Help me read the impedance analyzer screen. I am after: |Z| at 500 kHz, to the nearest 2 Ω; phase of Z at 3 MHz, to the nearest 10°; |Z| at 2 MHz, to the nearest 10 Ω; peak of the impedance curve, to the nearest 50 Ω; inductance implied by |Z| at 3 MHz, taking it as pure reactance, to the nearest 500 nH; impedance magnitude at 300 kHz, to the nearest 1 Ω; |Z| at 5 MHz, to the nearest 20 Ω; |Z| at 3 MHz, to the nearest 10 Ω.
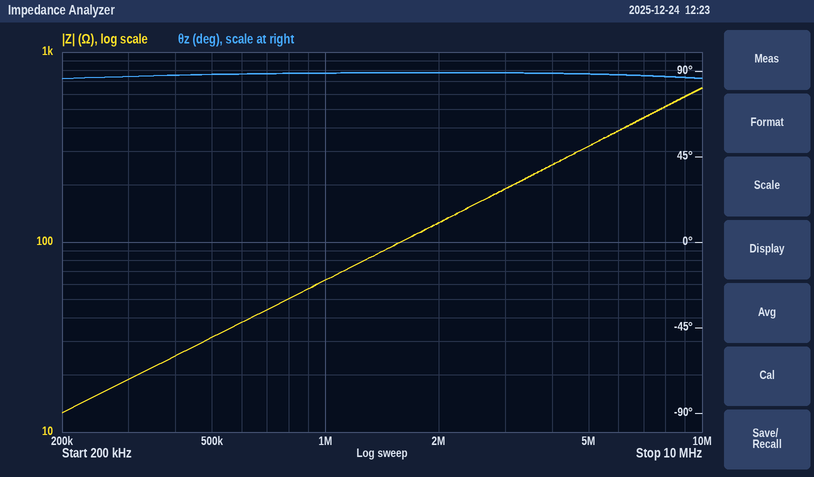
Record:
32 Ω
90°
130 Ω
650 Ω
10.0 µH
19 Ω
320 Ω
190 Ω
